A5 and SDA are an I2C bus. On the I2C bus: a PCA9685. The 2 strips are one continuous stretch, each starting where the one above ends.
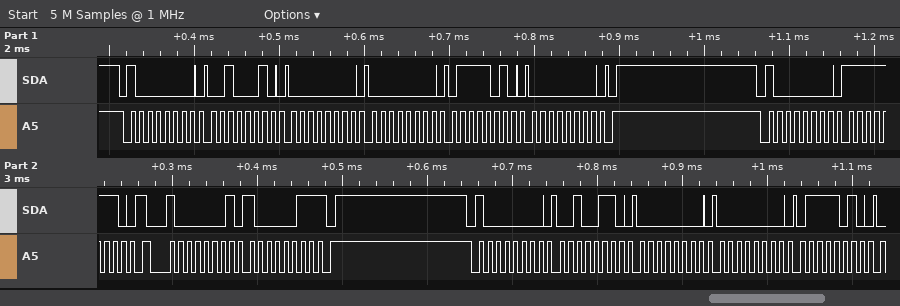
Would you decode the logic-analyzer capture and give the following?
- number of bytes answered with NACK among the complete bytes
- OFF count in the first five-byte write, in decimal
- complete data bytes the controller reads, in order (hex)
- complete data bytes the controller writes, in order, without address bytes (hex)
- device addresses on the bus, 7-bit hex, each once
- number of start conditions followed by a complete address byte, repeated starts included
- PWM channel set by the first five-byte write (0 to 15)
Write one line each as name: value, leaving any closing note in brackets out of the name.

number of bytes answered with NACK among the complete bytes: 1
OFF count in the first five-byte write, in decimal: 122
complete data bytes the controller reads, in order: 83
complete data bytes the controller writes, in order, without address bytes: 22 00 00 7A 00 FE 26 00 00 7A
device addresses on the bus, 7-bit hex, each once: 0x40
number of start conditions followed by a complete address byte, repeated starts included: 4
PWM channel set by the first five-byte write: 7
